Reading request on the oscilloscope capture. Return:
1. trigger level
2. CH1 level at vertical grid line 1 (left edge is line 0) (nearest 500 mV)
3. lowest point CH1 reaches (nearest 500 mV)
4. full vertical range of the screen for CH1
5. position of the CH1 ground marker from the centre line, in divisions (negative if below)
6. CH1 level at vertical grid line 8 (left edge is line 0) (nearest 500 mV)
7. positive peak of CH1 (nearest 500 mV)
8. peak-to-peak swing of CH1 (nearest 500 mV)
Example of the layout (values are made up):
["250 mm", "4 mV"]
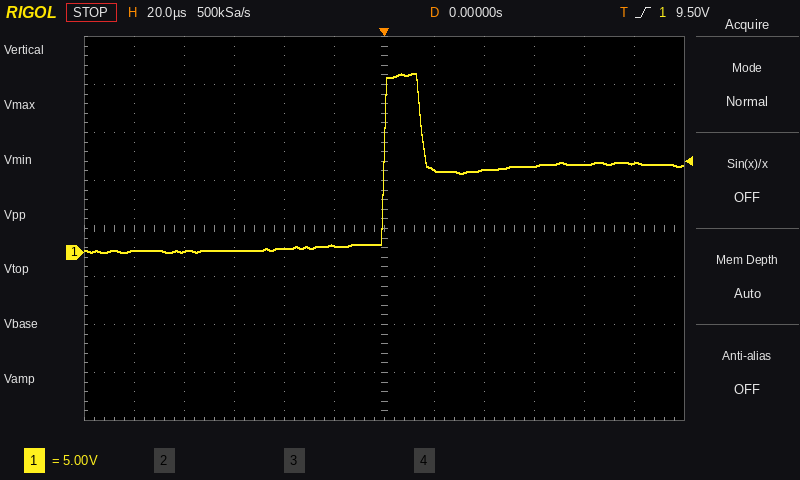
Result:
["9.50 V", "0.0 V", "0.0 V", "40 V", "-0.5 div", "8.5 V", "18.5 V", "18.5 V"]
